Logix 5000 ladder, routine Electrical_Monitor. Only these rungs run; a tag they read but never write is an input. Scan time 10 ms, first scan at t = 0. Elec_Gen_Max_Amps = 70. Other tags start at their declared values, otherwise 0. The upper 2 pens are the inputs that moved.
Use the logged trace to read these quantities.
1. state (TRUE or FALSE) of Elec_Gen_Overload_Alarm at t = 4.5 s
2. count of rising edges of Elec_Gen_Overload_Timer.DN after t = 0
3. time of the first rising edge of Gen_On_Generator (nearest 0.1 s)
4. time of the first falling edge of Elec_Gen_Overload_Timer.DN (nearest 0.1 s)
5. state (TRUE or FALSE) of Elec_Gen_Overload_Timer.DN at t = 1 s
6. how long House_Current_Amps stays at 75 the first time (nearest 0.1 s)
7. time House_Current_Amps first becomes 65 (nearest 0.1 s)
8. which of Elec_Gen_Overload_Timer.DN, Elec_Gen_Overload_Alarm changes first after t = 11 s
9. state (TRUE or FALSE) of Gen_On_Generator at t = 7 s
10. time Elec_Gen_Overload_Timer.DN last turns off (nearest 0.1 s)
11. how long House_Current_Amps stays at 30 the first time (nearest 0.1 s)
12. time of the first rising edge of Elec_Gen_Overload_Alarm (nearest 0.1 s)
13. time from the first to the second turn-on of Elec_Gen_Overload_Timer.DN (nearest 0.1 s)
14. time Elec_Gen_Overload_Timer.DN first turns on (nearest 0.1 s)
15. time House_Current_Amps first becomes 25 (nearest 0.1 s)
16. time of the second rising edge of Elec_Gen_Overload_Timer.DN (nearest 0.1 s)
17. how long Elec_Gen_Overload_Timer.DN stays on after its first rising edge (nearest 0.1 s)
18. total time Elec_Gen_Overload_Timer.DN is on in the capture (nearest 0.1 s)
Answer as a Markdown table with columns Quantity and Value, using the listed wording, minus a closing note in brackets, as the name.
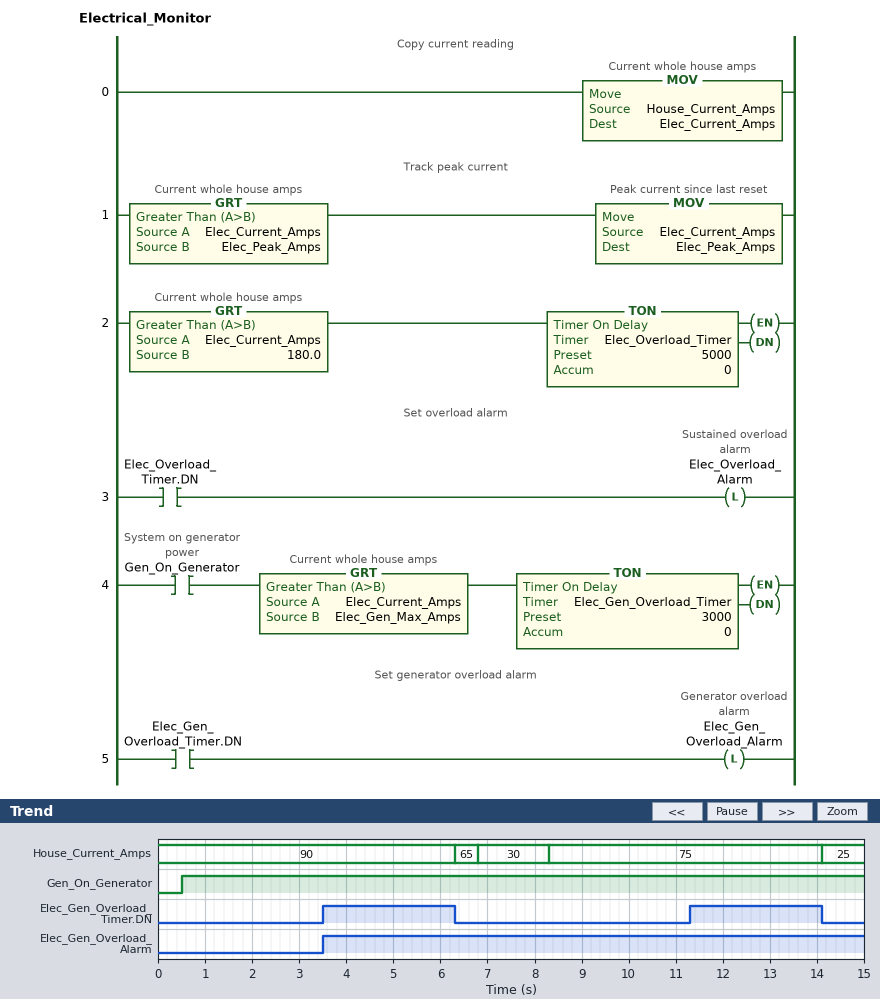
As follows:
| Quantity | Value |
|---|---|
| state (TRUE or FALSE) of Elec_Gen_Overload_Alarm at t = 4.5 s | TRUE |
| count of rising edges of Elec_Gen_Overload_Timer.DN after t = 0 | 2 |
| time of the first rising edge of Gen_On_Generator | 0.5 s |
| time of the first falling edge of Elec_Gen_Overload_Timer.DN | 6.3 s |
| state (TRUE or FALSE) of Elec_Gen_Overload_Timer.DN at t = 1 s | FALSE |
| how long House_Current_Amps stays at 75 the first time | 5.8 s |
| time House_Current_Amps first becomes 65 | 6.3 s |
| which of Elec_Gen_Overload_Timer.DN, Elec_Gen_Overload_Alarm changes first after t = 11 s | Elec_Gen_Overload_Timer.DN |
| state (TRUE or FALSE) of Gen_On_Generator at t = 7 s | TRUE |
| time Elec_Gen_Overload_Timer.DN last turns off | 14.1 s |
| how long House_Current_Amps stays at 30 the first time | 1.5 s |
| time of the first rising edge of Elec_Gen_Overload_Alarm | 3.5 s |
| time from the first to the second turn-on of Elec_Gen_Overload_Timer.DN | 7.8 s |
| time Elec_Gen_Overload_Timer.DN first turns on | 3.5 s |
| time House_Current_Amps first becomes 25 | 14.1 s |
| time of the second rising edge of Elec_Gen_Overload_Timer.DN | 11.3 s |
| how long Elec_Gen_Overload_Timer.DN stays on after its first rising edge | 2.8 s |
| total time Elec_Gen_Overload_Timer.DN is on in the capture | 5.6 s |
